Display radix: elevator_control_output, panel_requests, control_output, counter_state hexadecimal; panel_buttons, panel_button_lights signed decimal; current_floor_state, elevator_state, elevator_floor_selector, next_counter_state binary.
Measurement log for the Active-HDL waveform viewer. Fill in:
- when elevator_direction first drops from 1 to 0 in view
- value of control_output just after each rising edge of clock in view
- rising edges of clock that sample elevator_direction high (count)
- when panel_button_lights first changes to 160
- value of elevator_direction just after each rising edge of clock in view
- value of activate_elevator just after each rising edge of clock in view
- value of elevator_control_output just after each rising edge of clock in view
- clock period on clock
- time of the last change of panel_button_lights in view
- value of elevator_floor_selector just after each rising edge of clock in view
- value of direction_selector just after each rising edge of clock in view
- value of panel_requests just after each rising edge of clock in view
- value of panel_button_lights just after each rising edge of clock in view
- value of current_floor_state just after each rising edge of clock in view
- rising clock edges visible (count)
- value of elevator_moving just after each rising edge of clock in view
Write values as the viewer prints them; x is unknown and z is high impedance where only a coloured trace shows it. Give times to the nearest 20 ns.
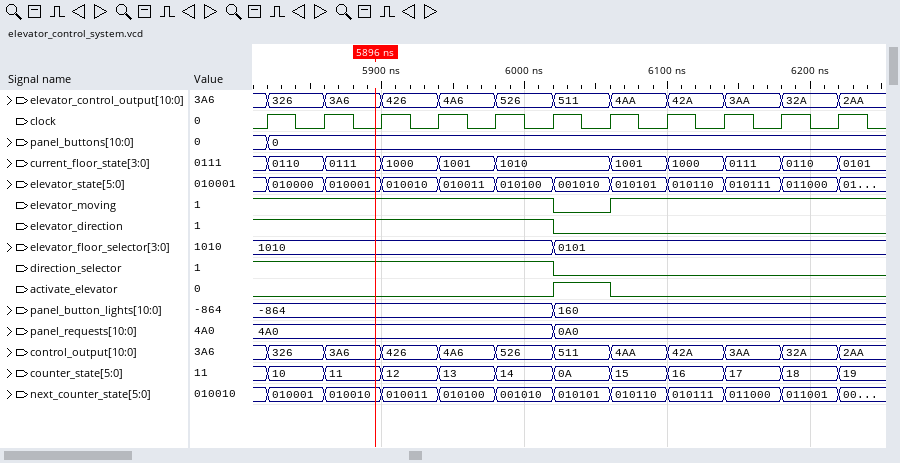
6020 ns
326, 3A6, 426, 4A6, 526, 511, 4AA, 42A, 3AA, 32A, 2AA
6
6020 ns
1 1 1 1 1 0 0 0 0 0 0
0 0 0 0 0 1 0 0 0 0 0
326, 3A6, 426, 4A6, 526, 511, 4AA, 42A, 3AA, 32A, 2AA
40 ns
6020 ns
1010, 1010, 1010, 1010, 1010, 0101, 0101, 0101, 0101, 0101, 0101
1 1 1 1 1 0 0 0 0 0 0
4A0, 4A0, 4A0, 4A0, 4A0, 0A0, 0A0, 0A0, 0A0, 0A0, 0A0
-864, -864, -864, -864, -864, 160, 160, 160, 160, 160, 160
0110, 0111, 1000, 1001, 1010, 1010, 1001, 1000, 0111, 0110, 0101
11
1 1 1 1 1 0 1 1 1 1 1
